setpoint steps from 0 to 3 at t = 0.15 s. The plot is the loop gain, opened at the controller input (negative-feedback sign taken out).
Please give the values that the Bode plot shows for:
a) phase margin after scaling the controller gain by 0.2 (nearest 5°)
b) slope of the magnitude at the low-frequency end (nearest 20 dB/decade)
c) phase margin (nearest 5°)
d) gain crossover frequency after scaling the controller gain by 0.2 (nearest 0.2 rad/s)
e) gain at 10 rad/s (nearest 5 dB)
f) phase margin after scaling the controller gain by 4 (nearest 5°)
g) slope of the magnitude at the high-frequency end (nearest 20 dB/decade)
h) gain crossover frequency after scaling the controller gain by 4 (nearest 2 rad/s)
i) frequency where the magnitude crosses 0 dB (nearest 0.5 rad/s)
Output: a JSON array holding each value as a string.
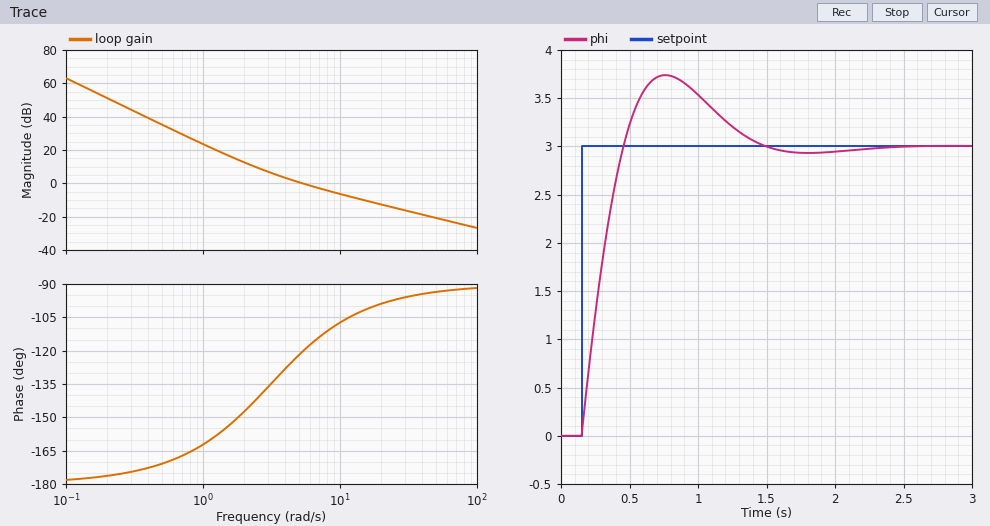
["30°", "-40 dB/decade", "60°", "1.8 rad/s", "-5 dB", "80°", "-20 dB/decade", "18 rad/s", "5.5 rad/s"]
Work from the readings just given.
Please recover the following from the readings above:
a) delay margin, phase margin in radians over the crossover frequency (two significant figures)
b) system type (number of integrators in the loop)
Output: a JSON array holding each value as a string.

["0.19 s", "2"]
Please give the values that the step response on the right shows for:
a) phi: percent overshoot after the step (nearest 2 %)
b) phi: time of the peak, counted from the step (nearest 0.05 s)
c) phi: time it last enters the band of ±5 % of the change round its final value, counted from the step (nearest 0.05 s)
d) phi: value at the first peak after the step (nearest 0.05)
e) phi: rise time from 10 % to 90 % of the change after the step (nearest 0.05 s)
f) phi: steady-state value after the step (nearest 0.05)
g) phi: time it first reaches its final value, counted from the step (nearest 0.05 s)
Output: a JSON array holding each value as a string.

["24 %", "0.60 s", "1.15 s", "3.75", "0.25 s", "3.00", "0.30 s"]
